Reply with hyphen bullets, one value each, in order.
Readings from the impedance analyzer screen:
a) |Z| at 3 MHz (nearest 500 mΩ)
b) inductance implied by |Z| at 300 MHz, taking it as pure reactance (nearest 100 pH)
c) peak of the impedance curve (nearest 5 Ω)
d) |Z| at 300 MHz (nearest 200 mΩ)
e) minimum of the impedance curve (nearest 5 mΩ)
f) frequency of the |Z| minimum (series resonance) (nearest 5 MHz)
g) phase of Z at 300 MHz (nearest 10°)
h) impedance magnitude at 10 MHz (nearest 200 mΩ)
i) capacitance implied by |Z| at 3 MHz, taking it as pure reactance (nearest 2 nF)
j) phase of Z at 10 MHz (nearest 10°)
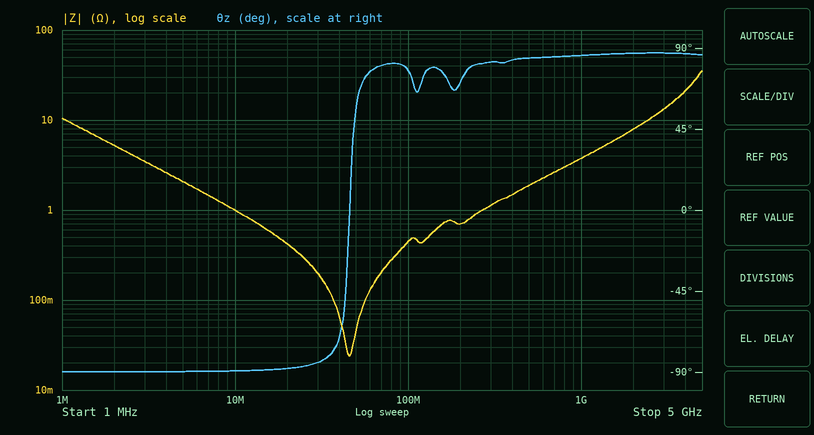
- 3.5 Ω
- 600 pH
- 35 Ω
- 1.2 Ω
- 25 mΩ
- 45 MHz
- 80°
- 1.0 Ω
- 16 nF
- -90°
